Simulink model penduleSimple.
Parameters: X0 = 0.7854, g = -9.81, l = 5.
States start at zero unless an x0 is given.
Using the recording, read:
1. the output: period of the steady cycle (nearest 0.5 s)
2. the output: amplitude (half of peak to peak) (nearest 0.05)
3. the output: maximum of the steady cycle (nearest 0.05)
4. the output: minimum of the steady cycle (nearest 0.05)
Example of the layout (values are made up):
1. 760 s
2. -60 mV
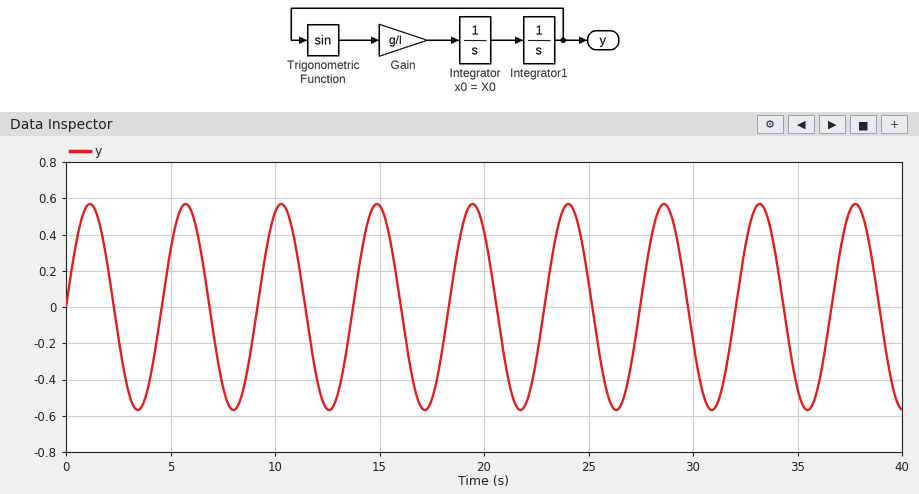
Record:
1. 4.5 s
2. 0.55
3. 0.55
4. -0.55
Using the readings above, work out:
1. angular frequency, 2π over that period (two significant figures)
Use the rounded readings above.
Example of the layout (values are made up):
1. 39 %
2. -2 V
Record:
1. 1.4 rad/s
